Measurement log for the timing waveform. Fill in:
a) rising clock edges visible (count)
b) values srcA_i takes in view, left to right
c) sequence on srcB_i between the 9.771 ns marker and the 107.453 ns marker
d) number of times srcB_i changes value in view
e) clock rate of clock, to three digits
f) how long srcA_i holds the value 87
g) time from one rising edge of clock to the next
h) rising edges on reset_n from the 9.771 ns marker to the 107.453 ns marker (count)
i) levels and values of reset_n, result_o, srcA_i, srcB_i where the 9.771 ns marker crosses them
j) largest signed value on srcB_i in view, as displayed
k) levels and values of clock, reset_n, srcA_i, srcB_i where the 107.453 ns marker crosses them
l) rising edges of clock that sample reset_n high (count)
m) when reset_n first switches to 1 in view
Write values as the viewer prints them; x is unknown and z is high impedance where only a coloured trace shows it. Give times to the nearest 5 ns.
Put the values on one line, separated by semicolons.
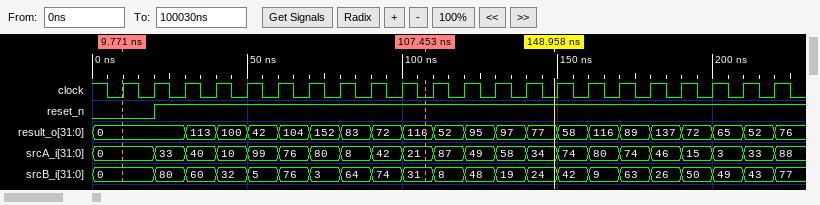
22; 0, 33, 40, 10, 99, 76, 80, 8, 42, 21, 87, 49, 58, 34, 74, 80, 74, 46, 15, 3, 33, 88; 0, 80, 60, 32, 5, 76, 3, 64, 74, 31; 21; 100 MHz; 10 ns; 10 ns; 1; reset_n=0, result_o=0, srcA_i=0, srcB_i=0; 80; clock=0, reset_n=1, srcA_i=21, srcB_i=31; 20; 20 ns
